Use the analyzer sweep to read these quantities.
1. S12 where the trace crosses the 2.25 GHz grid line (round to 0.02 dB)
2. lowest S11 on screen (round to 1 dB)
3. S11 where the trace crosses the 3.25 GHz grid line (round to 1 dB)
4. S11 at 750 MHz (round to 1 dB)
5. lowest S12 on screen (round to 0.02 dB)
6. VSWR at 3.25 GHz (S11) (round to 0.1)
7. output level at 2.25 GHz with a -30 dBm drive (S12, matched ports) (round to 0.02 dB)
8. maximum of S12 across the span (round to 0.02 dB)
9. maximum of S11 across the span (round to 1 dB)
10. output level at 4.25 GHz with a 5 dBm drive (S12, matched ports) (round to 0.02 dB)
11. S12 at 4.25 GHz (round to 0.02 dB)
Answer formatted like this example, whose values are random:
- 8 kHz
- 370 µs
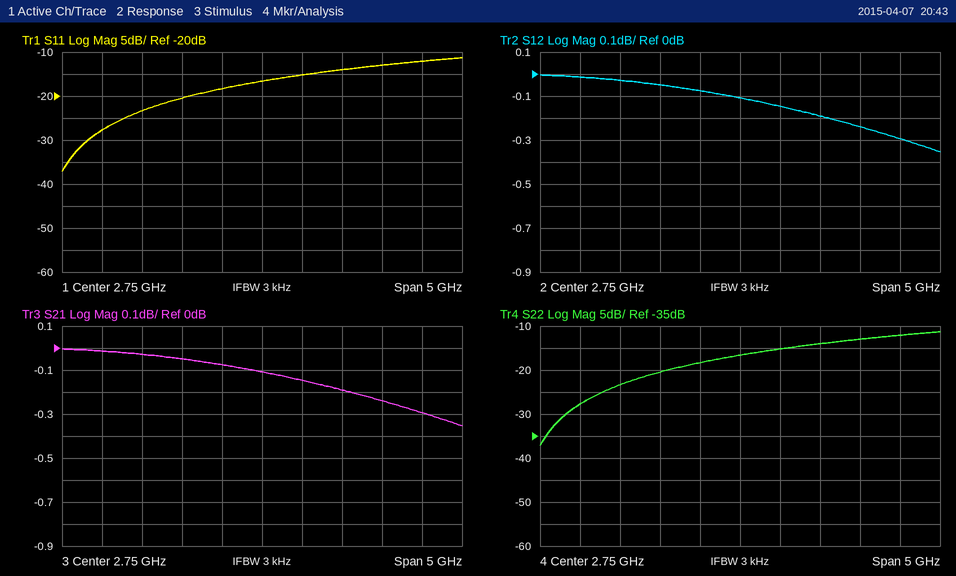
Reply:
- -0.08 dB
- -37 dB
- -15 dB
- -28 dB
- -0.36 dB
- 1.4
- -30.08 dBm
- 0.00 dB
- -11 dB
- 4.76 dBm
- -0.24 dB
